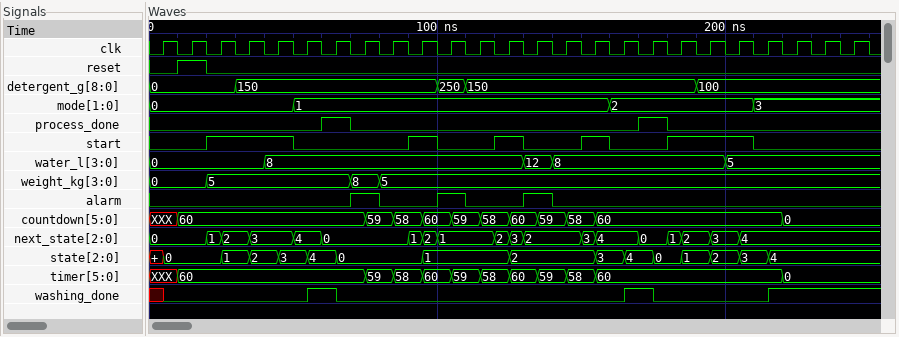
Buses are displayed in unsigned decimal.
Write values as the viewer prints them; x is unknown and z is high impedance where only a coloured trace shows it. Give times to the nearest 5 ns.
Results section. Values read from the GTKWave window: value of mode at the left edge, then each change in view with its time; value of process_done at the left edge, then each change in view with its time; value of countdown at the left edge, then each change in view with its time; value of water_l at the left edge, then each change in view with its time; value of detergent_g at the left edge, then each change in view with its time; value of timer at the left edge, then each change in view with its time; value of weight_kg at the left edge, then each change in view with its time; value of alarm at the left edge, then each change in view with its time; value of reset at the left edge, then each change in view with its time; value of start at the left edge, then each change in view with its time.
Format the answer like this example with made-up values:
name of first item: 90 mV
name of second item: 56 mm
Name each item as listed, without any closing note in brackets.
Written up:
value of mode at the left edge, then each change in view with its time: 0, 1 at 50 ns, 2 at 160 ns, 3 at 210 ns
value of process_done at the left edge, then each change in view with its time: 0, 1 at 60 ns, 0 at 70 ns, 1 at 170 ns, 0 at 180 ns
value of countdown at the left edge, then each change in view with its time: XXX, 60 at 10 ns, 59 at 75 ns, 58 at 85 ns, 60 at 95 ns, 59 at 105 ns, 58 at 115 ns, 60 at 125 ns, 59 at 135 ns, 58 at 145 ns, 60 at 155 ns, 0 at 220 ns
value of water_l at the left edge, then each change in view with its time: 0, 8 at 40 ns, 12 at 130 ns, 8 at 140 ns, 5 at 200 ns
value of detergent_g at the left edge, then each change in view with its time: 0, 150 at 30 ns, 250 at 100 ns, 150 at 110 ns, 100 at 190 ns
value of timer at the left edge, then each change in view with its time: XXX, 60 at 10 ns, 59 at 75 ns, 58 at 85 ns, 60 at 95 ns, 59 at 105 ns, 58 at 115 ns, 60 at 125 ns, 59 at 135 ns, 58 at 145 ns, 60 at 155 ns, 0 at 220 ns
value of weight_kg at the left edge, then each change in view with its time: 0, 5 at 20 ns, 8 at 70 ns, 5 at 80 ns
value of alarm at the left edge, then each change in view with its time: 0, 1 at 70 ns, 0 at 80 ns, 1 at 100 ns, 0 at 110 ns, 1 at 130 ns, 0 at 140 ns
value of reset at the left edge, then each change in view with its time: 0, 1 at 10 ns, 0 at 20 ns
value of start at the left edge, then each change in view with its time: 0, 1 at 20 ns, 0 at 50 ns, 1 at 90 ns, 0 at 100 ns, 1 at 120 ns, 0 at 130 ns, 1 at 150 ns, 0 at 160 ns, 1 at 180 ns, 0 at 210 ns
